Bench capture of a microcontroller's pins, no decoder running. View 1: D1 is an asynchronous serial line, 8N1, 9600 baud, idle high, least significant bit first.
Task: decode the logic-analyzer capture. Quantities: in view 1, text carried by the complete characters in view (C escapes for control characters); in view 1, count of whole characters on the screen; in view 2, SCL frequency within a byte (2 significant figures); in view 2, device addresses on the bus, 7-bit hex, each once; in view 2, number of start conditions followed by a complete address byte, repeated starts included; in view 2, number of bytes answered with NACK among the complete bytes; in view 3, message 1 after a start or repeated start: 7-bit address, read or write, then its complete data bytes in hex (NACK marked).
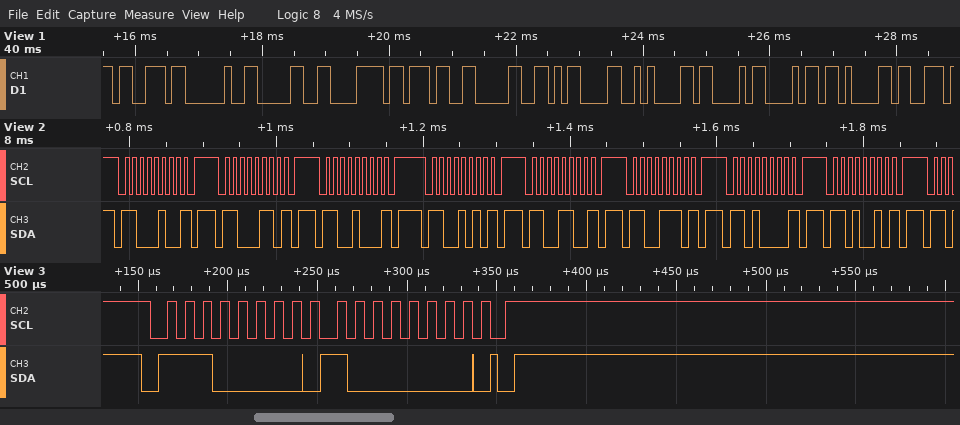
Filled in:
"s 0x70\r\nCha"
11
100 kHz
0x62 0x63 0x64 0x65 0x66 0x67 0x68 0x69
8
8
0x70 write: 80
